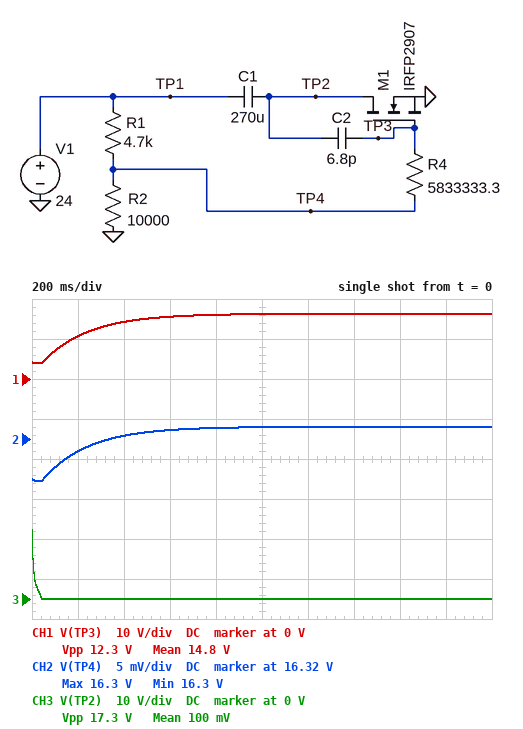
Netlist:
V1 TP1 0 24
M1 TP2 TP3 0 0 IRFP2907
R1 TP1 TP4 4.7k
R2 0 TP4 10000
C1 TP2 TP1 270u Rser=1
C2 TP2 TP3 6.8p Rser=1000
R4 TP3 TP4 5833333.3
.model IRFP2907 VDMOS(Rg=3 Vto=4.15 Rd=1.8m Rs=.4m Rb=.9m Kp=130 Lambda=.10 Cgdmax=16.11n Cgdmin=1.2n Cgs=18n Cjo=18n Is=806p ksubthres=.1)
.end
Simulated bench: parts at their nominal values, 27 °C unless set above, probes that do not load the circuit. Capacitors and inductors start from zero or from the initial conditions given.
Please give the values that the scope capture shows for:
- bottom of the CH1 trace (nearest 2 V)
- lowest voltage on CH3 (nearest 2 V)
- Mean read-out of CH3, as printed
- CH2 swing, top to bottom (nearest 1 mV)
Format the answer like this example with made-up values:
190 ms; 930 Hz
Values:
4 V; 0 V; 100 mV; 7 mV
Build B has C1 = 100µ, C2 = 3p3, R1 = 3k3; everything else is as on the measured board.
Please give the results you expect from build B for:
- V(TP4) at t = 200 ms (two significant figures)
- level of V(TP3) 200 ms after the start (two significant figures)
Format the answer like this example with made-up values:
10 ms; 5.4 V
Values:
18 V; 12 V
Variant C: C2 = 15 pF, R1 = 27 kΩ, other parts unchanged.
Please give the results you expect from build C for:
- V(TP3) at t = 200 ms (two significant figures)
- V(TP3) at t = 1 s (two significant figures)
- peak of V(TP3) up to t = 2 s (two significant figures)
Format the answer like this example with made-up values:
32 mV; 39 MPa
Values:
3.9 V; 6.4 V; 6.5 V
